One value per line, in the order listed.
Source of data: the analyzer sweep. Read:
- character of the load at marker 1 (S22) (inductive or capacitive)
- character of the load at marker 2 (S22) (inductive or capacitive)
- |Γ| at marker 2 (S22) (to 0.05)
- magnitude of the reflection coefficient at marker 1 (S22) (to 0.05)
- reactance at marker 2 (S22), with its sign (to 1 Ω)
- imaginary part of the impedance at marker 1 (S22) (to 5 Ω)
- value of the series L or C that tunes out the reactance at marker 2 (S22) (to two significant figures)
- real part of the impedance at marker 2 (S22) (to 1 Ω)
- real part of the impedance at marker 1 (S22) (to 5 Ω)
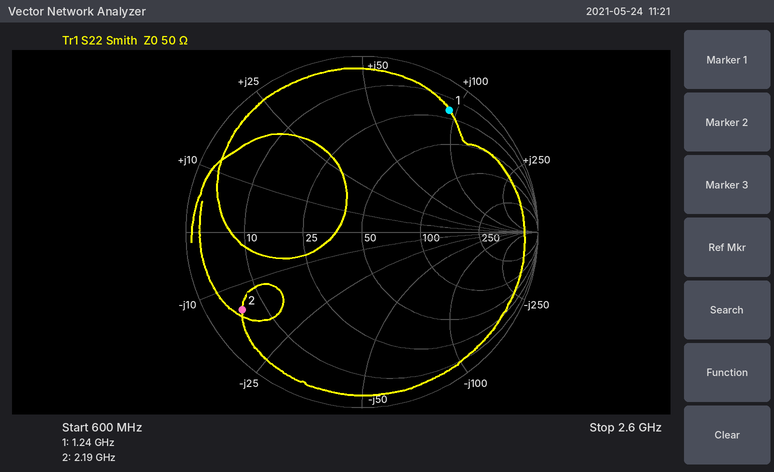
inductive
capacitive
0.80
0.85
-15 Ω
+95 Ω
1.1 nH
6 Ω
20 Ω
